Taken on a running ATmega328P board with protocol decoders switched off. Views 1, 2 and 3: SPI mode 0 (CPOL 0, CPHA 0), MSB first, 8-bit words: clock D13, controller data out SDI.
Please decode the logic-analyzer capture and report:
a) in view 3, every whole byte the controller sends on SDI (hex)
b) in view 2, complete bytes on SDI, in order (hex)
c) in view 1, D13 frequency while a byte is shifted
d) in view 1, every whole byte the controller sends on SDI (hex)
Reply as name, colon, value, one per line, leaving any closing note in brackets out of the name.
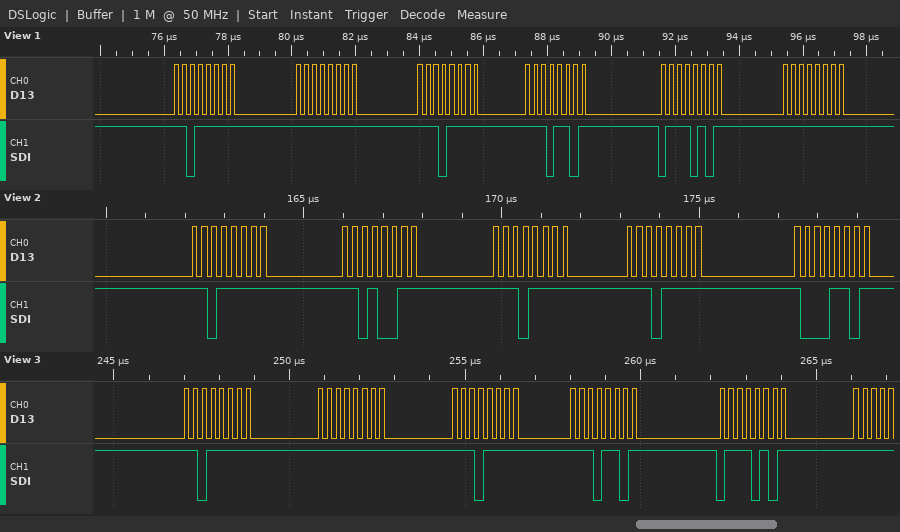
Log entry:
in view 3, every whole byte the controller sends on SDI: DF FF EF ED 75
in view 2, complete bytes on SDI, in order: DF D3 EF EF 8D
in view 1, D13 frequency while a byte is shifted: 4 MHz
in view 1, every whole byte the controller sends on SDI: DF FF EF ED 75 FF
